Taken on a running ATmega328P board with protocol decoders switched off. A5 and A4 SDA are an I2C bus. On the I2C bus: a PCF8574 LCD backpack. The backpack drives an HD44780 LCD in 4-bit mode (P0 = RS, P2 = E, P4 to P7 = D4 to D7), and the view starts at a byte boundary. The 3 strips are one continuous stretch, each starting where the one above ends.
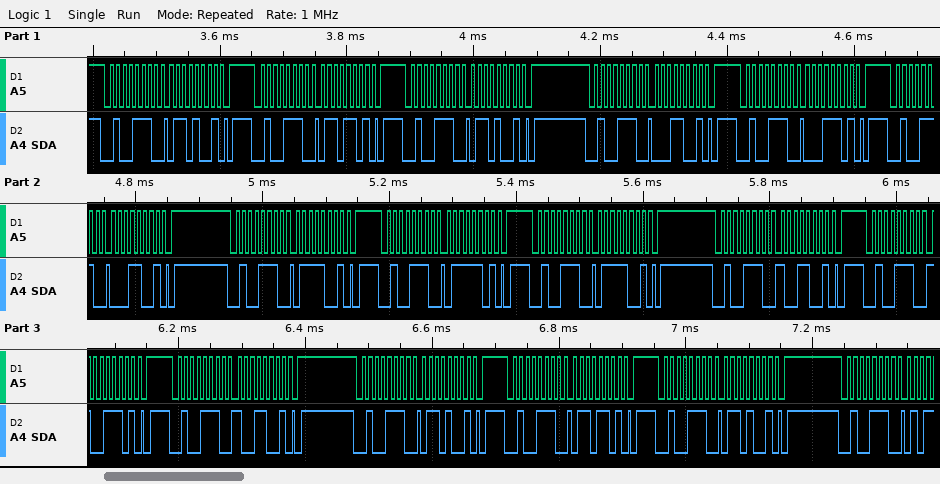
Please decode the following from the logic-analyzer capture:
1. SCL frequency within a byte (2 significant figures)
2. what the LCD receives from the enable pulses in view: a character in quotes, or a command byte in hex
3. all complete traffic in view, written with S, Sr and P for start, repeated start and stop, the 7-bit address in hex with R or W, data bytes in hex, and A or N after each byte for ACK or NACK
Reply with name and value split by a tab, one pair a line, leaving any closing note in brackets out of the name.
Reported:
SCL frequency within a byte	100 kHz
what the LCD receives from the enable pulses in view: a character in quotes, or a command byte in hex	'a' 'y'
all complete traffic in view, written with S, Sr and P for start, repeated start and stop, the 7-bit address in hex with R or W, data bytes in hex, and A or N after each byte for ACK or NACK	S 27W A 69 A P S 27W A 6D A P S 27W A 69 A P S 27W A 19 A P S 27W A 1D A P S 27W A 19 A P S 27W A 79 A P S 27W A 7D A P S 27W A 79 A P S 27W A 99 A P S 27W A 9D A P S 27W A 99 A P S 27W A 69 A P S 27W A 6D A P S 27W A 69 A P S 27W A
